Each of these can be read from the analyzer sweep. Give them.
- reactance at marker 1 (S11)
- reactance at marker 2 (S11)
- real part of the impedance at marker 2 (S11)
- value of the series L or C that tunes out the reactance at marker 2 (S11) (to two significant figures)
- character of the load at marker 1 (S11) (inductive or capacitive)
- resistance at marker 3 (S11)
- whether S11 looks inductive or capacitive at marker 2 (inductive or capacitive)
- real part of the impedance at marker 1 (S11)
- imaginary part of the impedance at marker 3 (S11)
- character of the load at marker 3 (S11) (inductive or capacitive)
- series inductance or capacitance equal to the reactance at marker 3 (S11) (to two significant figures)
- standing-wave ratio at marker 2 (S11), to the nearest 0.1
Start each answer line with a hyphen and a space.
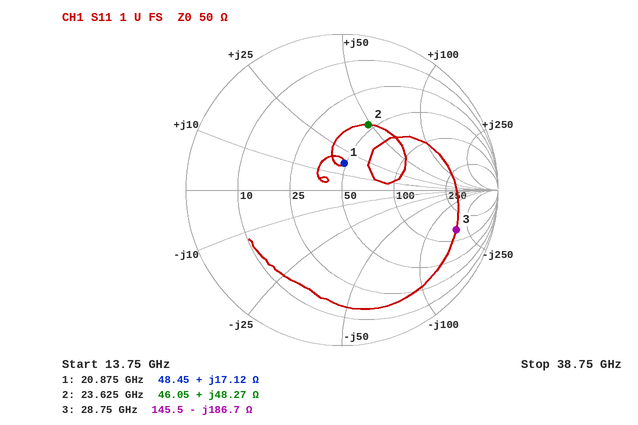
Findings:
- +17.12 Ω
- +48.27 Ω
- 46.05 Ω
- 140 fF
- inductive
- 145.5 Ω
- inductive
- 48.45 Ω
- -186.7 Ω
- capacitive
- 30 fF
- 2.6
